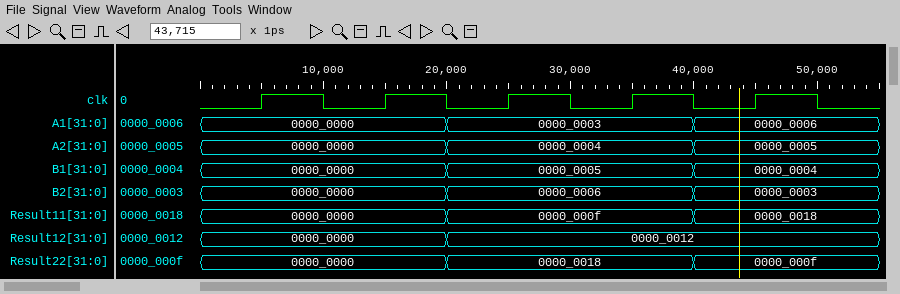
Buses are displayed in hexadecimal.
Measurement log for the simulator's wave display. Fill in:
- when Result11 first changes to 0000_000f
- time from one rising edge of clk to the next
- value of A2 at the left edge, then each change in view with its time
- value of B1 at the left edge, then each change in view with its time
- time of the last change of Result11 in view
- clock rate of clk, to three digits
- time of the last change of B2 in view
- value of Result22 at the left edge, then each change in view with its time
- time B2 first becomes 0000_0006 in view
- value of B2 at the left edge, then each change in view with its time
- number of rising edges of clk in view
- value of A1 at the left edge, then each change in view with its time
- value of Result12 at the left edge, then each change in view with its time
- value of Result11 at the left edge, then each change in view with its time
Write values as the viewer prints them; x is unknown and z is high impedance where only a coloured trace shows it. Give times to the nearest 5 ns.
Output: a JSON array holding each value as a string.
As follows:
["20 ns", "10 ns", "0000_0000, 0000_0004 at 20 ns, 0000_0005 at 40 ns", "0000_0000, 0000_0005 at 20 ns, 0000_0004 at 40 ns", "40 ns", "100 MHz", "40 ns", "0000_0000, 0000_0018 at 20 ns, 0000_000f at 40 ns", "20 ns", "0000_0000, 0000_0006 at 20 ns, 0000_0003 at 40 ns", "5", "0000_0000, 0000_0003 at 20 ns, 0000_0006 at 40 ns", "0000_0000, 0000_0012 at 20 ns", "0000_0000, 0000_000f at 20 ns, 0000_0018 at 40 ns"]
